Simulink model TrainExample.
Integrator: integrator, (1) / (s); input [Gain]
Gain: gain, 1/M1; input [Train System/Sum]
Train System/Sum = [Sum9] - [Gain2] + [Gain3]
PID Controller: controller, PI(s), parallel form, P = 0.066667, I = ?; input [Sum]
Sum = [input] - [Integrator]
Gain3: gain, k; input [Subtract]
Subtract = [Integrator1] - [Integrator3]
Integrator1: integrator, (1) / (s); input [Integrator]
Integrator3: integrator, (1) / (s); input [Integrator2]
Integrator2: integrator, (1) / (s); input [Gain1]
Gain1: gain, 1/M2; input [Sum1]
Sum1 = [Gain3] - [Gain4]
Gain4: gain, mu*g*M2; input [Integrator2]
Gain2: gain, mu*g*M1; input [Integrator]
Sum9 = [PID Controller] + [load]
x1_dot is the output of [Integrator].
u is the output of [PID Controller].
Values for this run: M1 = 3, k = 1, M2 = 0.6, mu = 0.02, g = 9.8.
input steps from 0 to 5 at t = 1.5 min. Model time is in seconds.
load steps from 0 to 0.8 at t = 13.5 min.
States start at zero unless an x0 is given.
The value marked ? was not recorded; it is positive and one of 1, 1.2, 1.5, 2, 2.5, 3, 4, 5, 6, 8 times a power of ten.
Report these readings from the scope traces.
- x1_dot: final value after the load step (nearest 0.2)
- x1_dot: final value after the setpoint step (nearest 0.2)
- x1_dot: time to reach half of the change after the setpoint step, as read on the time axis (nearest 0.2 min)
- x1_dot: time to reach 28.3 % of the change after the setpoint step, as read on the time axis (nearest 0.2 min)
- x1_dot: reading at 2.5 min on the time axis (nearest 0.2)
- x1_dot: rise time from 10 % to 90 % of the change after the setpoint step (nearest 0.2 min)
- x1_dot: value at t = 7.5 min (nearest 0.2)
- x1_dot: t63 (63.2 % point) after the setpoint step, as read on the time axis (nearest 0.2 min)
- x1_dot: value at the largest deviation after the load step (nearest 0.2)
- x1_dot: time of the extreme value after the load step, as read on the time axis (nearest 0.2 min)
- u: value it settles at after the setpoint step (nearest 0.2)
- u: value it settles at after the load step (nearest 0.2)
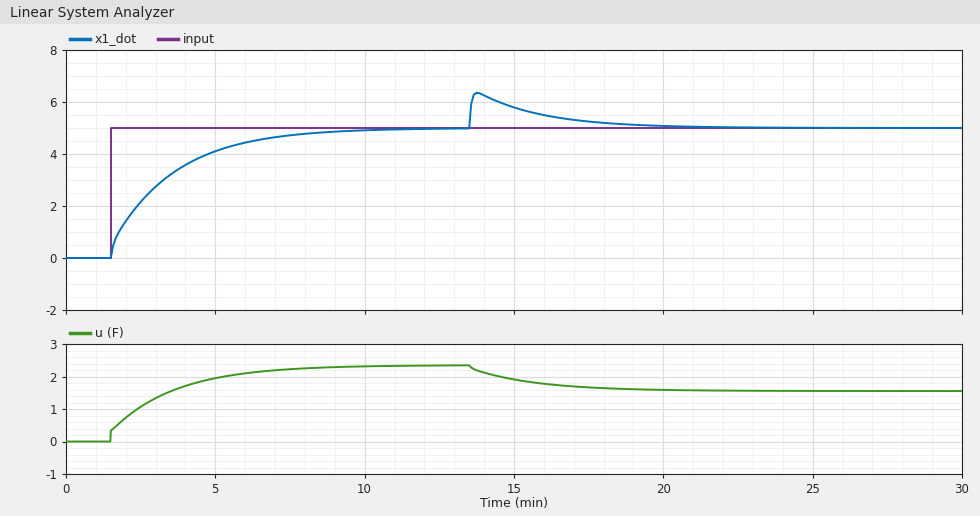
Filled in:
5.0
5.0
2.8 min
2.0 min
2.2
4.6 min
4.8
3.4 min
6.4
13.8 min
2.4
1.6
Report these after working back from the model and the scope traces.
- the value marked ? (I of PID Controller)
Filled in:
0.004
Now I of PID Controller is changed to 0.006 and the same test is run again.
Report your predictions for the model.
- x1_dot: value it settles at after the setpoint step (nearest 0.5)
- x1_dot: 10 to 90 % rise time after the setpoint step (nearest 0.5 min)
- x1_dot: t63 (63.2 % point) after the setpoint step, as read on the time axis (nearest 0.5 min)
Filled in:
5.0
3.0 min
3.0 min
